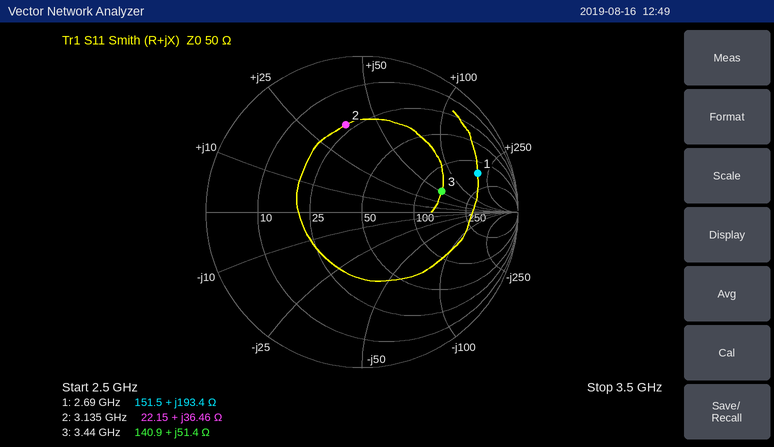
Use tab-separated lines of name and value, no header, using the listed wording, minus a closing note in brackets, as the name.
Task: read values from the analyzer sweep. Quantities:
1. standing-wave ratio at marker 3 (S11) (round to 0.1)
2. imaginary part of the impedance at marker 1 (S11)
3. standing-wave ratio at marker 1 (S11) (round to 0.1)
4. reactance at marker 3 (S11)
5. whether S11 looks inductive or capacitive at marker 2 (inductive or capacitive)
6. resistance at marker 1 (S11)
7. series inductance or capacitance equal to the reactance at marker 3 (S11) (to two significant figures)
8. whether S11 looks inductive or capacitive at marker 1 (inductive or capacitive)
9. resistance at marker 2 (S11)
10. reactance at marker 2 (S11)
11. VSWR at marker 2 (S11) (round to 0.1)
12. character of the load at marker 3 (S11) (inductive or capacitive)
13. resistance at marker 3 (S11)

standing-wave ratio at marker 3 (S11)	3.2
imaginary part of the impedance at marker 1	+193.4 Ω
standing-wave ratio at marker 1 (S11)	8.2
reactance at marker 3	+51.4 Ω
whether S11 looks inductive or capacitive at marker 2	inductive
resistance at marker 1	151.5 Ω
series inductance or capacitance equal to the reactance at marker 3 (S11)	2.4 nH
whether S11 looks inductive or capacitive at marker 1	inductive
resistance at marker 2	22.15 Ω
reactance at marker 2	+36.46 Ω
VSWR at marker 2 (S11)	3.6
character of the load at marker 3 (S11)	inductive
resistance at marker 3	140.9 Ω
